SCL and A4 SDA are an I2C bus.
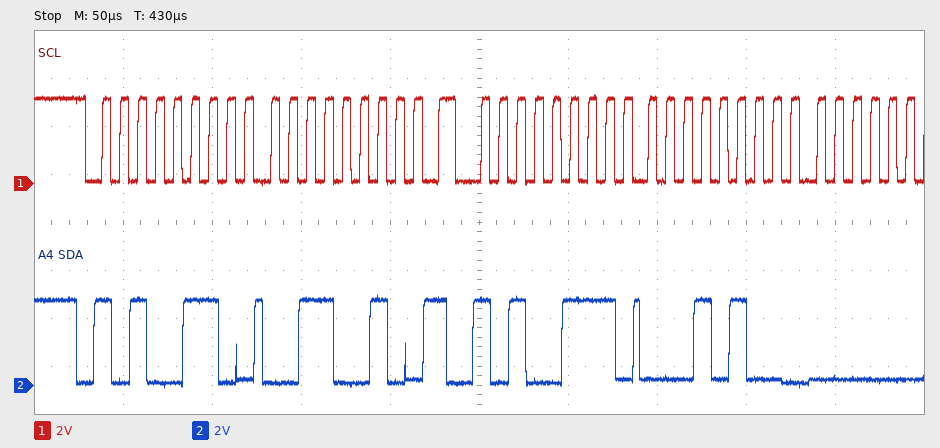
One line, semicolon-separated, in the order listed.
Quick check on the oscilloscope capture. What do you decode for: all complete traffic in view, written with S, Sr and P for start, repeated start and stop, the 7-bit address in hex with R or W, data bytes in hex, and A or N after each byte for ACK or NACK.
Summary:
S 53W A 32 A Sr 53R A 14 A
